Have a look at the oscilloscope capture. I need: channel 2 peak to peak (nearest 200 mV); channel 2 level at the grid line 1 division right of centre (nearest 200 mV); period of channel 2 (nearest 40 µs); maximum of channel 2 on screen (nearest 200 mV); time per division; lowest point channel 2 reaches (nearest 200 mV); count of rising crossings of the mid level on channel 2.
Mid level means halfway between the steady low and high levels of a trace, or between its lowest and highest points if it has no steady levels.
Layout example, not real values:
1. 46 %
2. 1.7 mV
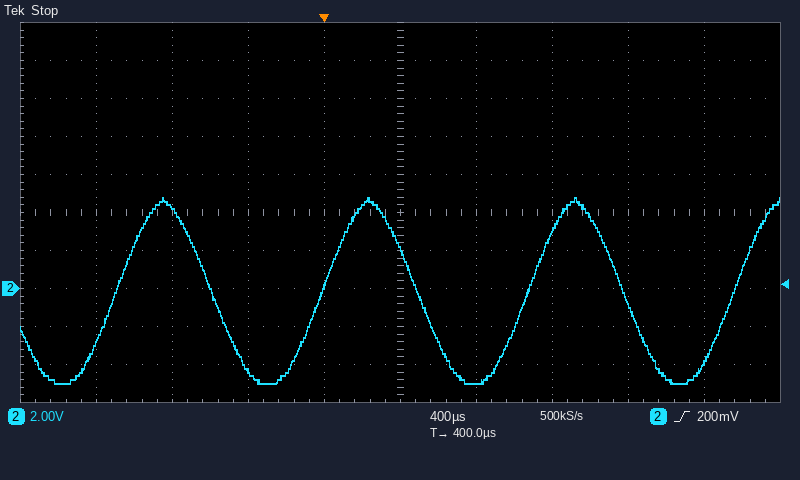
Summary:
1. 9.8 V
2. -5.0 V
3. 1.08 ms
4. 4.8 V
5. 400 µs
6. -5.0 V
7. 4
